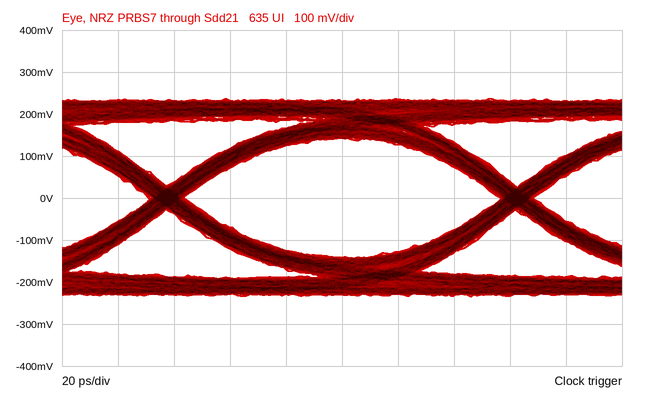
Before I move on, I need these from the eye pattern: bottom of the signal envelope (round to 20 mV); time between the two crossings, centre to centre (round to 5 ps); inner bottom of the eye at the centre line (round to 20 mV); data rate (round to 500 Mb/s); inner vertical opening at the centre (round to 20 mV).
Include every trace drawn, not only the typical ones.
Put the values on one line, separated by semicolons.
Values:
-240 mV; 125 ps; -140 mV; 8.0 Gb/s; 280 mV
